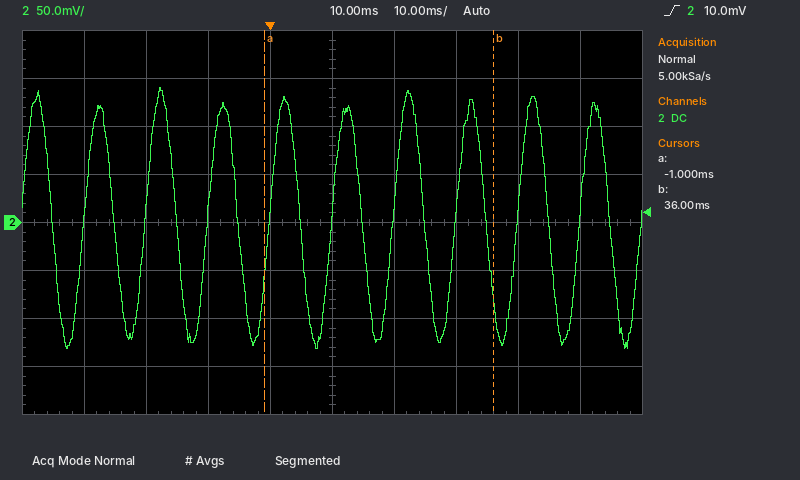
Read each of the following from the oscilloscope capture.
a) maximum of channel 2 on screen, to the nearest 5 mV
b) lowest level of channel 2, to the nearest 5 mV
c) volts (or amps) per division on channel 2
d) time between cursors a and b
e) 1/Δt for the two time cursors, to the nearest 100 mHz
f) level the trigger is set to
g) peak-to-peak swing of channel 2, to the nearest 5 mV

140 mV
-130 mV
50 mV
37 ms
27.0 Hz
10.0 mV
270 mV
